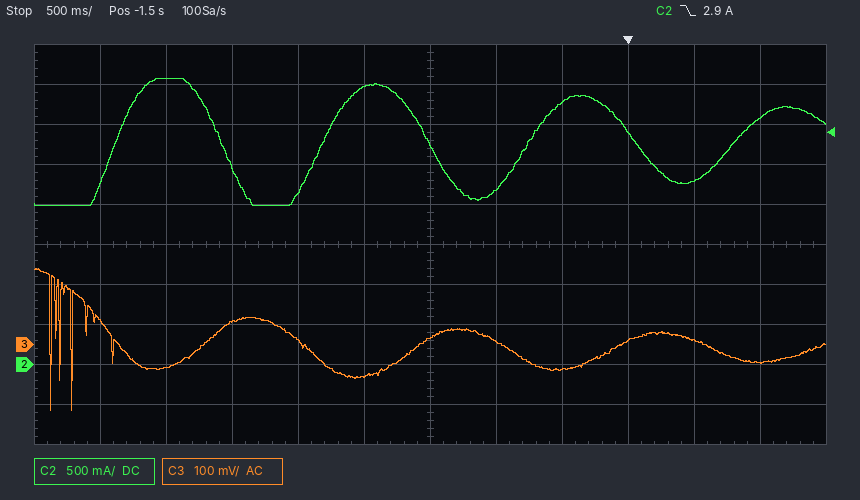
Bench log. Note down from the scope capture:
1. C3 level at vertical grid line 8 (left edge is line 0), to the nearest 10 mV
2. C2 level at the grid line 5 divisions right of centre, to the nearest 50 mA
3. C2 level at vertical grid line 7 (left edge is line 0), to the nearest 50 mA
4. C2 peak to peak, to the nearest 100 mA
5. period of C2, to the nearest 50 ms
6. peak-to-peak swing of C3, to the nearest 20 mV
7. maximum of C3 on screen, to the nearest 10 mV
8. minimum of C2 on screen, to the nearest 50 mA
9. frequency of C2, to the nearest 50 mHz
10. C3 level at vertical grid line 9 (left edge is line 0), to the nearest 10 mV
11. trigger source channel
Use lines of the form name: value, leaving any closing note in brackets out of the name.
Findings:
C3 level at vertical grid line 8 (left edge is line 0), to the nearest 10 mV: -60 mV
C2 level at the grid line 5 divisions right of centre, to the nearest 50 mA: 3.10 A
C2 level at vertical grid line 7 (left edge is line 0), to the nearest 50 mA: 2.20 A
C2 peak to peak, to the nearest 100 mA: 1.60 A
period of C2, to the nearest 50 ms: 1.55 s
peak-to-peak swing of C3, to the nearest 20 mV: 360 mV
maximum of C3 on screen, to the nearest 10 mV: 190 mV
minimum of C2 on screen, to the nearest 50 mA: 2.00 A
frequency of C2, to the nearest 50 mHz: 650 mHz
C3 level at vertical grid line 9 (left edge is line 0), to the nearest 10 mV: 10 mV
trigger source channel: C2
